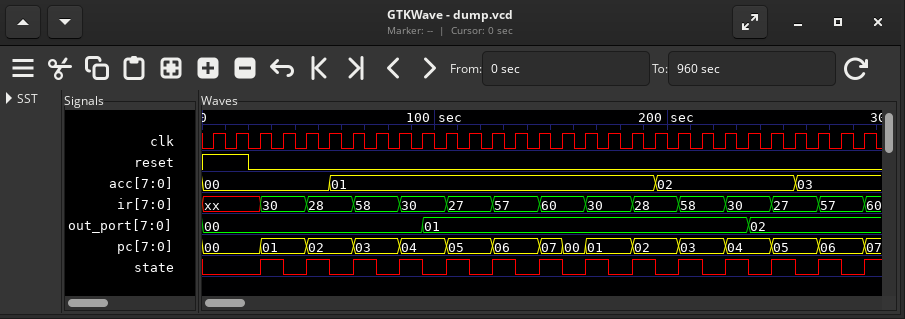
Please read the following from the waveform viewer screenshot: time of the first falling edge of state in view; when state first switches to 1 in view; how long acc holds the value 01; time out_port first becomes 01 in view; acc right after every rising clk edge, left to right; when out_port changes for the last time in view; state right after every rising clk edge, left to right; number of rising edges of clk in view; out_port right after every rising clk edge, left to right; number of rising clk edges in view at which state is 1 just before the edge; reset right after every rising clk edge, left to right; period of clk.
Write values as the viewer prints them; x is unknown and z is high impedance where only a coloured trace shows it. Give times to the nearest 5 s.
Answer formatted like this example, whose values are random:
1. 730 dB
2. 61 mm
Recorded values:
1. 35 s
2. 25 s
3. 140 s
4. 95 s
5. 00, 00, 00, 00, 00, 01, 01, 01, 01, 01, 01, 01, 01, 01, 01, 01, 01, 01, 01, 02, 02, 02, 02, 02, 02, 03, 03, 03, 03
6. 235 s
7. 0 0 1 0 1 0 1 0 1 0 1 0 1 0 1 0 1 0 1 0 1 0 1 0 1 0 1 0 1
8. 29
9. 00, 00, 00, 00, 00, 00, 00, 00, 00, 01, 01, 01, 01, 01, 01, 01, 01, 01, 01, 01, 01, 01, 01, 02, 02, 02, 02, 02, 02
10. 13
11. 1 1 0 0 0 0 0 0 0 0 0 0 0 0 0 0 0 0 0 0 0 0 0 0 0 0 0 0 0
12. 10 s
